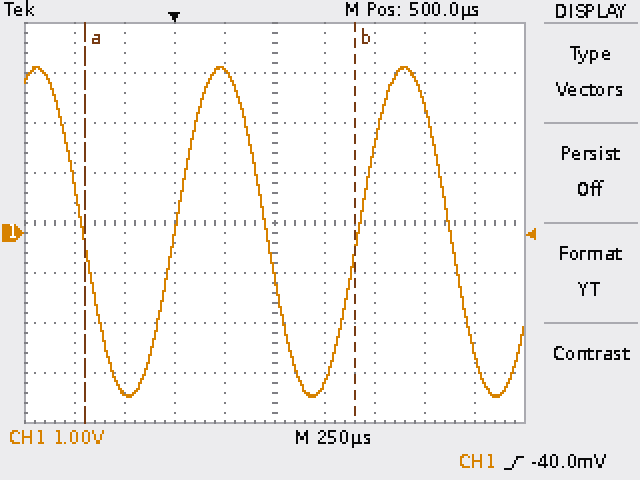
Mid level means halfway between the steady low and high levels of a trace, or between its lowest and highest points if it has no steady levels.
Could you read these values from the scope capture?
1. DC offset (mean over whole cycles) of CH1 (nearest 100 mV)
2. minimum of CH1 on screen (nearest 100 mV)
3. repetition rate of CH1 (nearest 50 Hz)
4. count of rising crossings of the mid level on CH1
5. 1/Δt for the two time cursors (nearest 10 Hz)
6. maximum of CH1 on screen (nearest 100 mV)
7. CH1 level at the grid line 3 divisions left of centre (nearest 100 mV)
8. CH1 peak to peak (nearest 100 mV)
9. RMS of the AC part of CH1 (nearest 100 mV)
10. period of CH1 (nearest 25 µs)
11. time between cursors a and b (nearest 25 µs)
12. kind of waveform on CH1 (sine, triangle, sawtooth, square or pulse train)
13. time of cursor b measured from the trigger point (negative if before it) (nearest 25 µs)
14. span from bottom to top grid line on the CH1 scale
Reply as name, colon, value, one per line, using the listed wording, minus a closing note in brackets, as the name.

DC offset (mean over whole cycles) of CH1: 0.0 V
minimum of CH1 on screen: -3.3 V
repetition rate of CH1: 1.10 kHz
count of rising crossings of the mid level on CH1: 2
1/Δt for the two time cursors: 740 Hz
maximum of CH1 on screen: 3.3 V
CH1 level at the grid line 3 divisions left of centre: -3.2 V
CH1 peak to peak: 6.6 V
RMS of the AC part of CH1: 2.3 V
period of CH1: 925 µs
time between cursors a and b: 1.350 ms
kind of waveform on CH1: sine
time of cursor b measured from the trigger point (negative if before it): +900 µs
span from bottom to top grid line on the CH1 scale: 8 V
